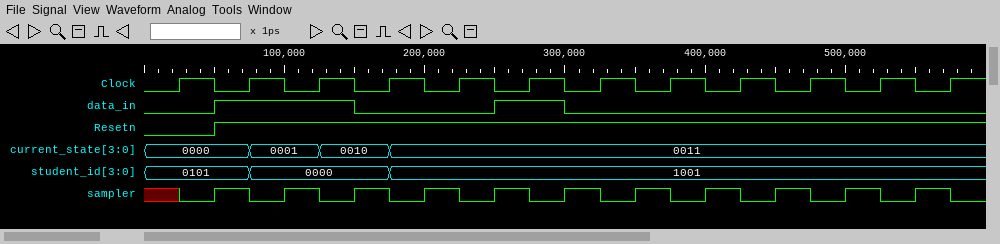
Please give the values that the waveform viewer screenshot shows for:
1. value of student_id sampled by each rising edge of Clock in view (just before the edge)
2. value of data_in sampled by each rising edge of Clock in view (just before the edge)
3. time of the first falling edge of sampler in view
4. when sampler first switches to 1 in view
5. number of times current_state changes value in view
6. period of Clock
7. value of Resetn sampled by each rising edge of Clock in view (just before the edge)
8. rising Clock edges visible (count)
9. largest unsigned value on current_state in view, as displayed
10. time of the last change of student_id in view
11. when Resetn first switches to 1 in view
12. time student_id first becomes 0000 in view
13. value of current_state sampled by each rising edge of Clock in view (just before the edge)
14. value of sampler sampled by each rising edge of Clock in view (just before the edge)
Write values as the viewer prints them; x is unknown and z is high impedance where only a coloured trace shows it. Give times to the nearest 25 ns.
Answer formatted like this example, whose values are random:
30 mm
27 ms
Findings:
0101, 0101, 0000, 0000, 1001, 1001, 1001, 1001, 1001, 1001, 1001, 1001
0 1 1 0 0 1 0 0 0 0 0 0
75 ns
50 ns
3
50 ns
0 1 1 1 1 1 1 1 1 1 1 1
12
0011
175 ns
50 ns
75 ns
0000, 0000, 0001, 0010, 0011, 0011, 0011, 0011, 0011, 0011, 0011, 0011
x 1 1 1 1 1 1 1 1 1 1 1
